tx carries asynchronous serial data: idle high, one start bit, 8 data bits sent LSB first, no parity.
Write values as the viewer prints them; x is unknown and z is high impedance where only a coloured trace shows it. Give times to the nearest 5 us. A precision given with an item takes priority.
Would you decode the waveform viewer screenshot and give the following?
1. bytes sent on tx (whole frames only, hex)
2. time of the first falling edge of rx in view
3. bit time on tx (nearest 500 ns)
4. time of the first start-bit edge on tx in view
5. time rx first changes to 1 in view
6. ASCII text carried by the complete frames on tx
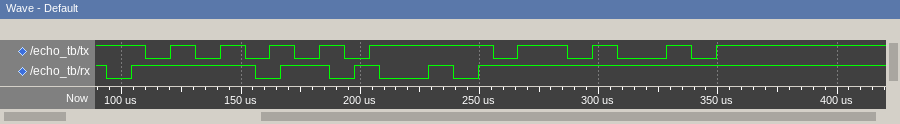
55, 4B
95 us
10500 ns
110 us
105 us
"UK"
